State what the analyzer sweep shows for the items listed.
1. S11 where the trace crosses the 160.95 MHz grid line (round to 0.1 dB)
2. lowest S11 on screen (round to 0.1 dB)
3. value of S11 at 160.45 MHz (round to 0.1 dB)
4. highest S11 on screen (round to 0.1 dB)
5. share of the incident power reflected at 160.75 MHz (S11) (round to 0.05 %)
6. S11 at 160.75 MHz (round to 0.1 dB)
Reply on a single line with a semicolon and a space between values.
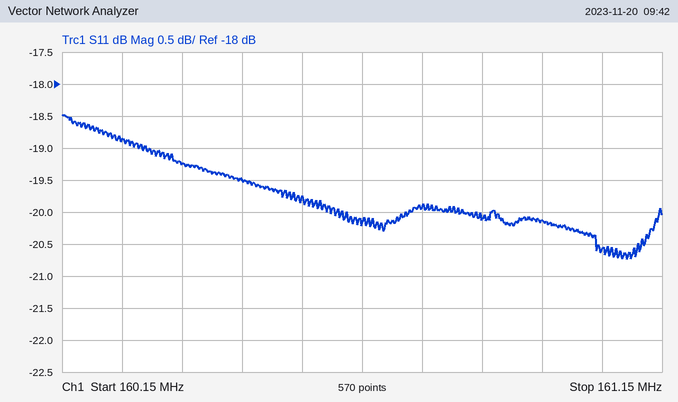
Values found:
-20.1 dB; -20.7 dB; -19.5 dB; -18.5 dB; 1.00 %; -19.9 dB
